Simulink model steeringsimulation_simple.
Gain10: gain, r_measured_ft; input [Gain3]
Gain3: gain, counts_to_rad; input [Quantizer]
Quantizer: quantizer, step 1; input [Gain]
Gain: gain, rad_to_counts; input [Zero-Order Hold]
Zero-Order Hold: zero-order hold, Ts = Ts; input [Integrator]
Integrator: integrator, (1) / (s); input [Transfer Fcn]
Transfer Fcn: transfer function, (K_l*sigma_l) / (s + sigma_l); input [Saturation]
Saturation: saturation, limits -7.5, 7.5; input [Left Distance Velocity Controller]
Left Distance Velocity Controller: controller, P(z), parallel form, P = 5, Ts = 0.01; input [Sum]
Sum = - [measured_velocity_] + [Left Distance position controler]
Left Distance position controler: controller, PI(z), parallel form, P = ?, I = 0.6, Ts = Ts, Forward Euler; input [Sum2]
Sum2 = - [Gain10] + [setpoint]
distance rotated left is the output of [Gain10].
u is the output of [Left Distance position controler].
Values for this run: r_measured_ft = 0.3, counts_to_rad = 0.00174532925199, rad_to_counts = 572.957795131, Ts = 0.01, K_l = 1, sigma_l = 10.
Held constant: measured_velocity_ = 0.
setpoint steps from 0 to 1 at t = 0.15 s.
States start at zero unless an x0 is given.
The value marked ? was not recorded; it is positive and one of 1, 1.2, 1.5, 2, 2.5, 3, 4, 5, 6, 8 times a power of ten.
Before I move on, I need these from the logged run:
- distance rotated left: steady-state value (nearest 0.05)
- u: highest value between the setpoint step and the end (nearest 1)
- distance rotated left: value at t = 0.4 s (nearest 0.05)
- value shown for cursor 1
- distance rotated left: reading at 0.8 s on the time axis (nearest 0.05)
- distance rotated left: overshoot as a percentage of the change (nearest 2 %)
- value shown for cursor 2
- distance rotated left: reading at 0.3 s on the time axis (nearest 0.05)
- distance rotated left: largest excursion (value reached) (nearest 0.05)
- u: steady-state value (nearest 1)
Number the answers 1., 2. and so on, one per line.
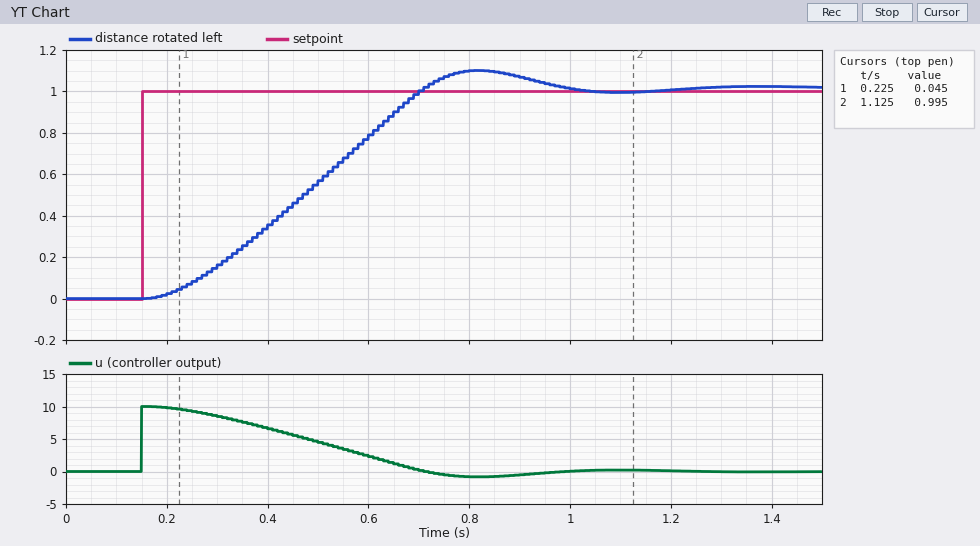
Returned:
1. 1.00
2. 10
3. 0.35
4. 0.045
5. 1.10
6. 8 %
7. 0.995
8. 0.15
9. 1.10
10. 0
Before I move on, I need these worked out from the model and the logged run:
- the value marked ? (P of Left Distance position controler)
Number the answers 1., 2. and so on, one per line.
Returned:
1. 10
